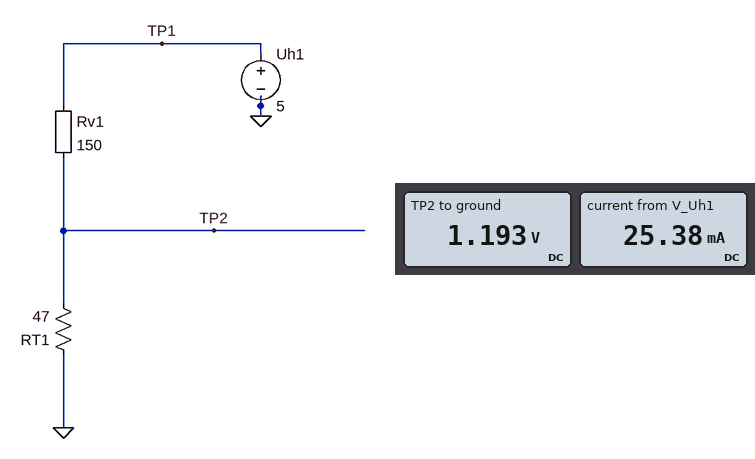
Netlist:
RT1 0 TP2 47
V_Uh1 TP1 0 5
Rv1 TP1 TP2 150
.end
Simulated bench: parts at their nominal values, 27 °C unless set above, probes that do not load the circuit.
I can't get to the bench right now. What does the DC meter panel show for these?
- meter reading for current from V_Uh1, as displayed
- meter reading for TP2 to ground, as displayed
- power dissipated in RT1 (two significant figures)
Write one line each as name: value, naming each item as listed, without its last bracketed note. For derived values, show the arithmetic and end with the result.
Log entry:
meter reading for current from V_Uh1, as displayed: 25.38 mA
meter reading for TP2 to ground, as displayed: 1.193 V
power dissipated in RT1: (1.193 V)^2 / 47 Ω = 30 mW
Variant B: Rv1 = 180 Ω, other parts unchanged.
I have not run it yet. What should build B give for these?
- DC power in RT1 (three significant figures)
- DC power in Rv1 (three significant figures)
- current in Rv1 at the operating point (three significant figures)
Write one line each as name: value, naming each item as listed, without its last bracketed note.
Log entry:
DC power in RT1: 22.8 mW
DC power in Rv1: 87.3 mW
current in Rv1 at the operating point: 22.0 mA
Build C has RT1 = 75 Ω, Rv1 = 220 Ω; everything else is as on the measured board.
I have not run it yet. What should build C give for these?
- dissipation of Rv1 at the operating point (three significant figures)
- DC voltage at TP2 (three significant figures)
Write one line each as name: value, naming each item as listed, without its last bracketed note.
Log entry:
dissipation of Rv1 at the operating point: 63.2 mW
DC voltage at TP2: 1.27 V
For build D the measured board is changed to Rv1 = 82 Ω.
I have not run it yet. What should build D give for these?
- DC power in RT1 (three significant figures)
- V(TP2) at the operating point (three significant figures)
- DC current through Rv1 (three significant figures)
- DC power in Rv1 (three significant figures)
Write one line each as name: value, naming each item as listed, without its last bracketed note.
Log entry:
DC power in RT1: 70.6 mW
V(TP2) at the operating point: 1.82 V
DC current through Rv1: 38.8 mA
DC power in Rv1: 123 mW
